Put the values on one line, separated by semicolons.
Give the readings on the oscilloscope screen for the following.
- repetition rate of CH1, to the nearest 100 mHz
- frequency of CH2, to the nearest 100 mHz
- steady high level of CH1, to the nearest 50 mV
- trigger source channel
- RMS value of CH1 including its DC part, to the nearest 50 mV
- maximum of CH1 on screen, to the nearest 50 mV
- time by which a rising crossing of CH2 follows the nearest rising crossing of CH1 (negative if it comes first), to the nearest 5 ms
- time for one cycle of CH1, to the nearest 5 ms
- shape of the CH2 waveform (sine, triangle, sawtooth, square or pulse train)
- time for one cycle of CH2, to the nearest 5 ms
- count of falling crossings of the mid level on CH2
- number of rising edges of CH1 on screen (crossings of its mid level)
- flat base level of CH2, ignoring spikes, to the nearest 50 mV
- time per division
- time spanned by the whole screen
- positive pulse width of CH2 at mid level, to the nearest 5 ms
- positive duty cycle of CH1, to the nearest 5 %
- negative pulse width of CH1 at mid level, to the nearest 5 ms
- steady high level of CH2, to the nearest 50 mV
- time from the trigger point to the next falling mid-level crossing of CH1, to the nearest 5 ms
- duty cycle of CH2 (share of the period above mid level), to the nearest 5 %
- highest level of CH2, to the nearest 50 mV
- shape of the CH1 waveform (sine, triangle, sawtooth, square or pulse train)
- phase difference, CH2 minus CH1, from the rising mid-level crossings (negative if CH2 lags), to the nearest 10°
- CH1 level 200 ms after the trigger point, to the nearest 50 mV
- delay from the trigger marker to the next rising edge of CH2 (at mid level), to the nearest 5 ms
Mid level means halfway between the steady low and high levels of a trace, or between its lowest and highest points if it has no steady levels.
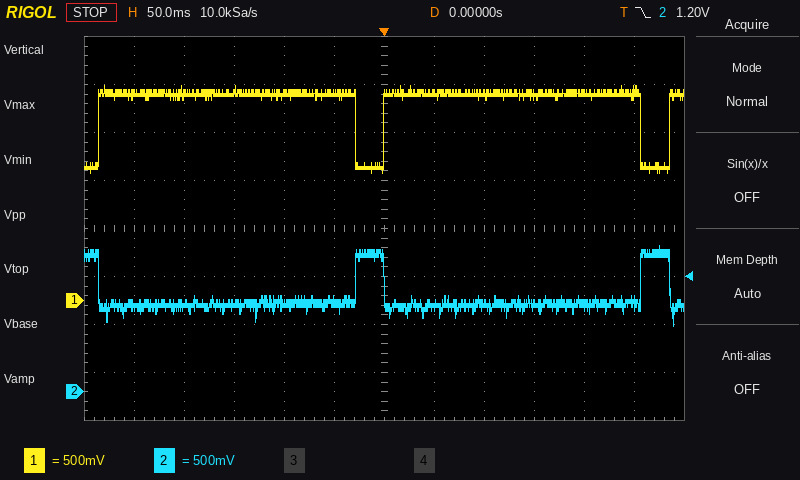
3.5 Hz; 3.5 Hz; 2.15 V; CH2; 2.10 V; 2.25 V; -30 ms; 285 ms; pulse train; 285 ms; 3; 3; 900 mV; 50 ms; 600 ms; 30 ms; 90 %; 30 ms; 1.45 V; 255 ms; 10 %; 1.50 V; pulse train; +40°; 2.15 V; 255 ms
